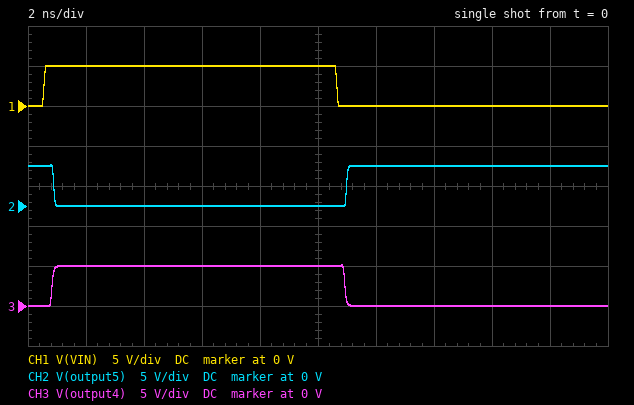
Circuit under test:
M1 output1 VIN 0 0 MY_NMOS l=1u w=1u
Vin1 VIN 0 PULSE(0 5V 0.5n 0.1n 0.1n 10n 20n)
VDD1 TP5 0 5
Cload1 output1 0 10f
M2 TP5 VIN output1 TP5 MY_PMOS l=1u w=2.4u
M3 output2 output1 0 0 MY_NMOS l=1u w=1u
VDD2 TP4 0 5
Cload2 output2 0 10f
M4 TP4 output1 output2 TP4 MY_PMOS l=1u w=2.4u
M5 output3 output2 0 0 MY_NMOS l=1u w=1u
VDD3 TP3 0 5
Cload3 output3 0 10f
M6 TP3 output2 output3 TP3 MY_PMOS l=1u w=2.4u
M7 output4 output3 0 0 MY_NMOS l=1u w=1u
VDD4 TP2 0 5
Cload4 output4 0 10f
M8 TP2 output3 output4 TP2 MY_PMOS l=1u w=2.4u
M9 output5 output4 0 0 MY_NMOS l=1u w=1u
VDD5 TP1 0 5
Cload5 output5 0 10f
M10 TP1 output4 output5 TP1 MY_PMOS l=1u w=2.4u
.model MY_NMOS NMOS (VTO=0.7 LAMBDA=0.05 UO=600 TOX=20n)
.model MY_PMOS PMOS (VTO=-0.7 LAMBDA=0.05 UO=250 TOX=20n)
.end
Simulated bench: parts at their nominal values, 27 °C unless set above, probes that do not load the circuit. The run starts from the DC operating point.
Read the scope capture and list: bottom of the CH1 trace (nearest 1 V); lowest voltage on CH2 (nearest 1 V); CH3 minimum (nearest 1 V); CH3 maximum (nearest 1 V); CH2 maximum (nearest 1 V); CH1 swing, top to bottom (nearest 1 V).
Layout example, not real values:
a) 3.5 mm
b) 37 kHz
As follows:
a) 0 V
b) 0 V
c) 0 V
d) 5 V
e) 5 V
f) 5 V
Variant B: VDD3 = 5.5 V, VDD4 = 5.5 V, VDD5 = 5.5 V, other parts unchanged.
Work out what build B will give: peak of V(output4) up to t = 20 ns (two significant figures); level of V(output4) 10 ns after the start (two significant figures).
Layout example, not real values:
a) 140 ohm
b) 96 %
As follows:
a) 5.6 V
b) 5.5 V
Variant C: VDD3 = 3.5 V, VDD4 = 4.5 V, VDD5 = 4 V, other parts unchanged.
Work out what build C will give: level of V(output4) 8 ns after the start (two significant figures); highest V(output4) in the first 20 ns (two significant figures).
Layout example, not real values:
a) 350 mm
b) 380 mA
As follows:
a) 4.5 V
b) 4.6 V
